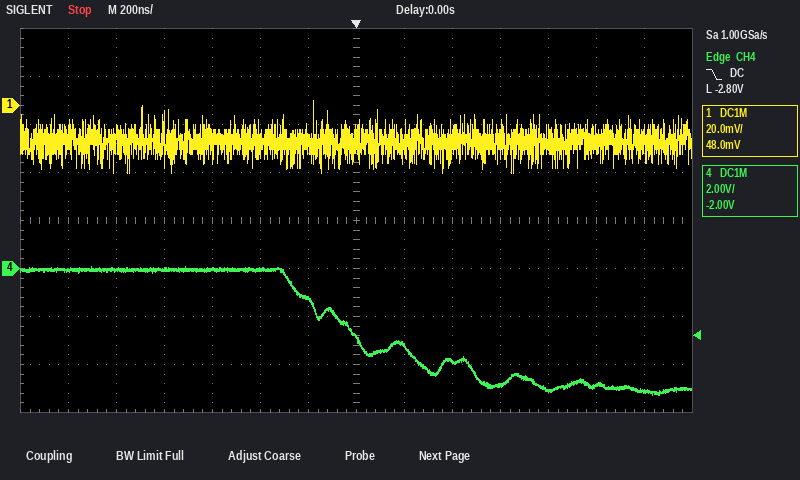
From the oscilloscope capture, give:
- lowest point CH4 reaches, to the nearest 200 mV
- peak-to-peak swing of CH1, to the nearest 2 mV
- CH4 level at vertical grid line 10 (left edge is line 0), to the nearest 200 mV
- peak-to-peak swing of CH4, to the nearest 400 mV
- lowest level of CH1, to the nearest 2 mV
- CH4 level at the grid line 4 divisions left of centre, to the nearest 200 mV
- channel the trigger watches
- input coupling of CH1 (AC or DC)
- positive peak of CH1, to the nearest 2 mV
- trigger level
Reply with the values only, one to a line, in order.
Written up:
-5.2 V
30 mV
-4.8 V
5.2 V
-28 mV
0.0 V
CH4
DC
2 mV
-2.80 V
